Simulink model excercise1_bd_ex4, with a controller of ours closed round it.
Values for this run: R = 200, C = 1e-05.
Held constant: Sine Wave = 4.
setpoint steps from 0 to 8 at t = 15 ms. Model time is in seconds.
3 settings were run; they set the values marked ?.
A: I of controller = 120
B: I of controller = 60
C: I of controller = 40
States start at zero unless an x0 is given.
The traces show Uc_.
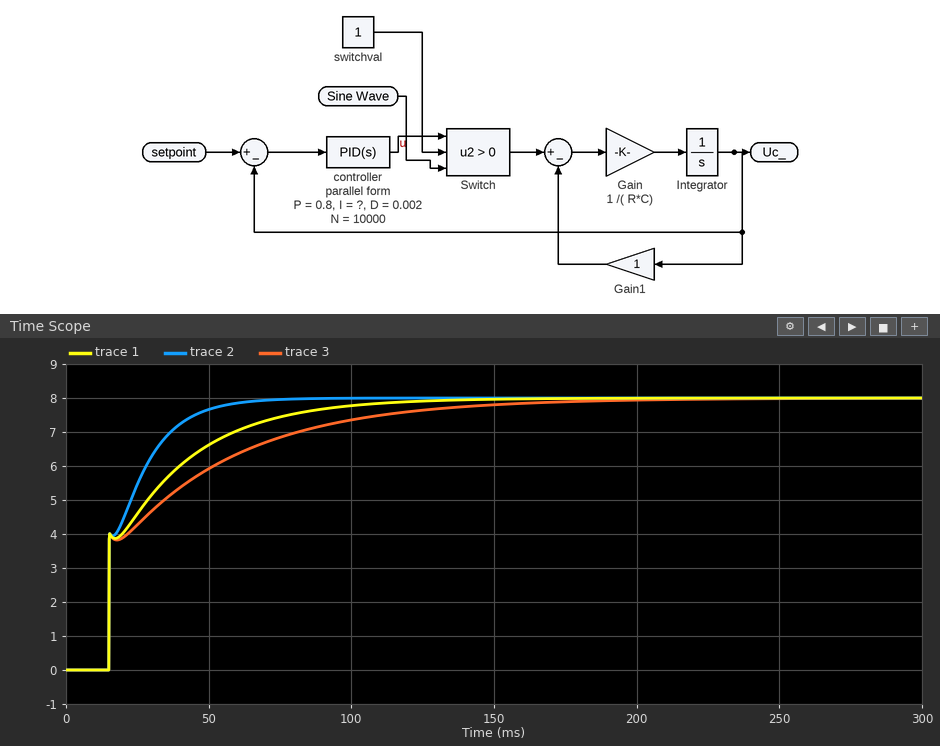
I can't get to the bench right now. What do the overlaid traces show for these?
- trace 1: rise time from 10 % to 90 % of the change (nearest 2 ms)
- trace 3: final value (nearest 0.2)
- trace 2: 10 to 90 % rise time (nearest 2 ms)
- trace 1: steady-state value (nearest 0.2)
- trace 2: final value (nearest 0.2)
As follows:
50 ms
8.0
24 ms
8.0
8.0
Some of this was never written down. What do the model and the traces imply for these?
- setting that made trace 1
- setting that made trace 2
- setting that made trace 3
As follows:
B
A
C
